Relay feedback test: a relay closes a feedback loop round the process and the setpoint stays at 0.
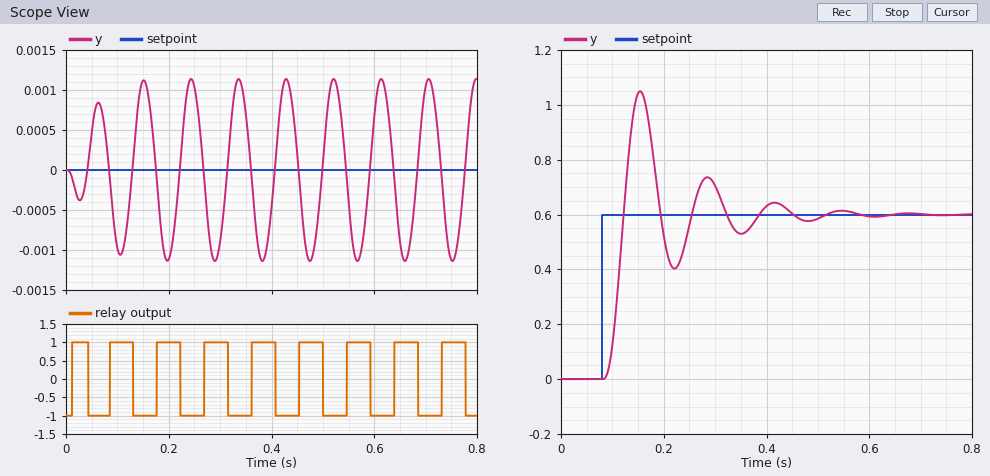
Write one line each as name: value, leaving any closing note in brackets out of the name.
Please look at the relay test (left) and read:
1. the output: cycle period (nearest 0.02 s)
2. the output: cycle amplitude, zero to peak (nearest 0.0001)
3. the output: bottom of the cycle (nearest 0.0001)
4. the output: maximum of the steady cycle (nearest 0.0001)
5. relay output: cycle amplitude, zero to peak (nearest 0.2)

the output: cycle period: 0.10 s
the output: cycle amplitude, zero to peak: 0.0011
the output: bottom of the cycle: -0.0011
the output: maximum of the steady cycle: 0.0011
relay output: cycle amplitude, zero to peak: 1.0
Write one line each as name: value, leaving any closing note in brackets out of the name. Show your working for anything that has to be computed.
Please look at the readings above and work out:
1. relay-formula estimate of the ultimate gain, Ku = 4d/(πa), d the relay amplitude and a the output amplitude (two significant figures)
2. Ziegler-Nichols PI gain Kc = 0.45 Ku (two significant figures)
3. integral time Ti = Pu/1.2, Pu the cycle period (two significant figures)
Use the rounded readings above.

relay-formula estimate of the ultimate gain, Ku = 4d/(πa), d the relay amplitude and a the output amplitude: 4 × 1 / (π × 0.0011) = 1200
Ziegler-Nichols PI gain Kc = 0.45 Ku: 0.45 × 1200 = 540
integral time Ti = Pu/1.2, Pu the cycle period: 0.1 / 1.2 = 0.083 s
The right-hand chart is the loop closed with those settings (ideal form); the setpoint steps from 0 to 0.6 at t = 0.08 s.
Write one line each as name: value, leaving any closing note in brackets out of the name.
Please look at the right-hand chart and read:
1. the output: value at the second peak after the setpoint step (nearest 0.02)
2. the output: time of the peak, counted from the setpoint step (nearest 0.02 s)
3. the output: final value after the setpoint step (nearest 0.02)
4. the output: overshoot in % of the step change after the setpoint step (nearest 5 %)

the output: value at the second peak after the setpoint step: 0.74
the output: time of the peak, counted from the setpoint step: 0.08 s
the output: final value after the setpoint step: 0.60
the output: overshoot in % of the step change after the setpoint step: 75 %
